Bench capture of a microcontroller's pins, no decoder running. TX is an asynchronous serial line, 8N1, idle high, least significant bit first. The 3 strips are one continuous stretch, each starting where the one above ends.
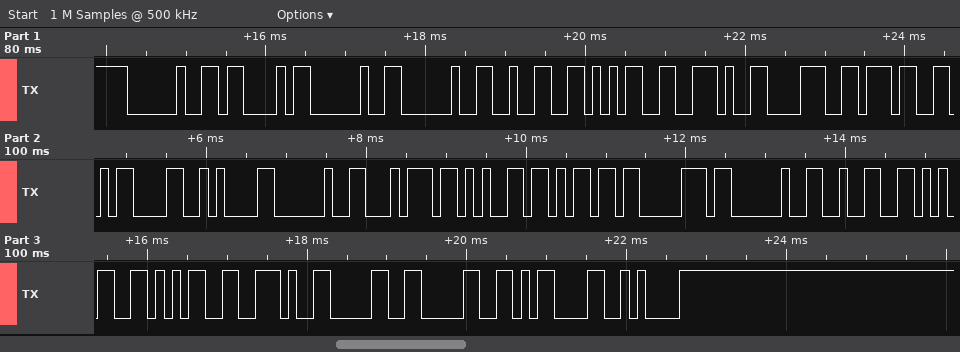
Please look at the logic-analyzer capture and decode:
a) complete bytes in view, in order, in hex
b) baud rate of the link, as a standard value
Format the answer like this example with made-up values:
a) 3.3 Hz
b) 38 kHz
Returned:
a) 20 43 20 20 32 35 2E 38 37 0D 0A 20 74 65 6D 70 20 32 35 35 2E 30 30 0D 0A
b) 9600 baud
